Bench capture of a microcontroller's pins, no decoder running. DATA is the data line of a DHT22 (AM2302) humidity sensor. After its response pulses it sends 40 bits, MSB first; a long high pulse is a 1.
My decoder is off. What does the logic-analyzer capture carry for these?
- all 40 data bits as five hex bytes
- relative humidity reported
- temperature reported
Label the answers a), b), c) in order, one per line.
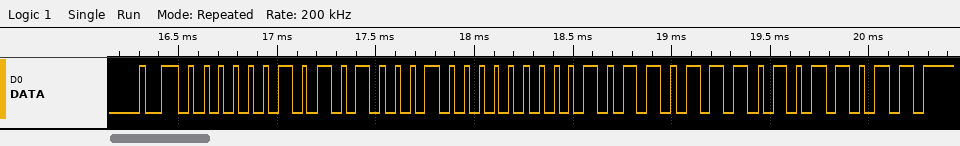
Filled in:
a) 02 A2 00 B7 5B
b) 67.4 %
c) 18.3 °C
